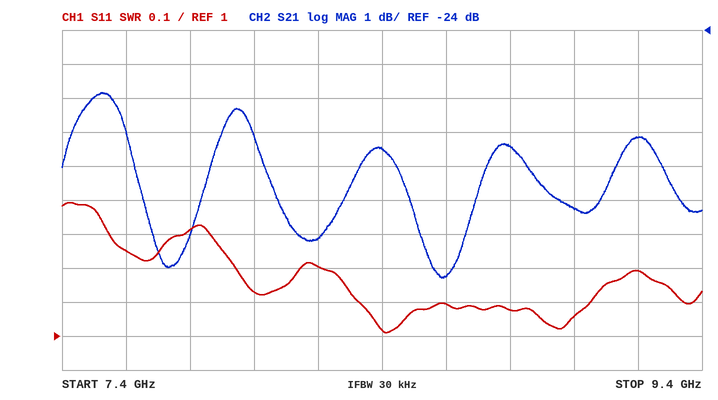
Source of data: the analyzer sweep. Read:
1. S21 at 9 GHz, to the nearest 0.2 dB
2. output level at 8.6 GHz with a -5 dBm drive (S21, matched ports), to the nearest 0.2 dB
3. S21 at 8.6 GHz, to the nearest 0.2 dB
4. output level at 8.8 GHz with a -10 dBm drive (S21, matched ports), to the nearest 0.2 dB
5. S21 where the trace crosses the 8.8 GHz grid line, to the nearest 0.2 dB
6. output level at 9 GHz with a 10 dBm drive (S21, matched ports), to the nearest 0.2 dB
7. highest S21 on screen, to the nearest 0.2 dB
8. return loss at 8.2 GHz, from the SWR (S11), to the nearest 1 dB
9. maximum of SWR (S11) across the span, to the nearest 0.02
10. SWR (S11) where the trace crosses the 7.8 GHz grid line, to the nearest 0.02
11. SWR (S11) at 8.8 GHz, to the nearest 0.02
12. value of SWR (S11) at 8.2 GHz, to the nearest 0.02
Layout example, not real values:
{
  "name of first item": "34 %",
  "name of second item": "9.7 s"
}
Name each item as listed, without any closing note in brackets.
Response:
{
  "S21 at 9 GHz, to the nearest 0.2 dB": "-29.2 dB",
  "output level at 8.6 GHz with a -5 dBm drive (S21, matched ports), to the nearest 0.2 dB": "-36.2 dBm",
  "S21 at 8.6 GHz, to the nearest 0.2 dB": "-31.2 dB",
  "output level at 8.8 GHz with a -10 dBm drive (S21, matched ports), to the nearest 0.2 dB": "-37.4 dBm",
  "S21 where the trace crosses the 8.8 GHz grid line, to the nearest 0.2 dB": "-27.4 dB",
  "output level at 9 GHz with a 10 dBm drive (S21, matched ports), to the nearest 0.2 dB": "-19.2 dBm",
  "highest S21 on screen, to the nearest 0.2 dB": "-25.8 dB",
  "return loss at 8.2 GHz, from the SWR (S11), to the nearest 1 dB": "21 dB",
  "maximum of SWR (S11) across the span, to the nearest 0.02": "1.40",
  "SWR (S11) where the trace crosses the 7.8 GHz grid line, to the nearest 0.02": "1.32",
  "SWR (S11) at 8.8 GHz, to the nearest 0.02": "1.08",
  "value of SWR (S11) at 8.2 GHz, to the nearest 0.02": "1.20"
}
